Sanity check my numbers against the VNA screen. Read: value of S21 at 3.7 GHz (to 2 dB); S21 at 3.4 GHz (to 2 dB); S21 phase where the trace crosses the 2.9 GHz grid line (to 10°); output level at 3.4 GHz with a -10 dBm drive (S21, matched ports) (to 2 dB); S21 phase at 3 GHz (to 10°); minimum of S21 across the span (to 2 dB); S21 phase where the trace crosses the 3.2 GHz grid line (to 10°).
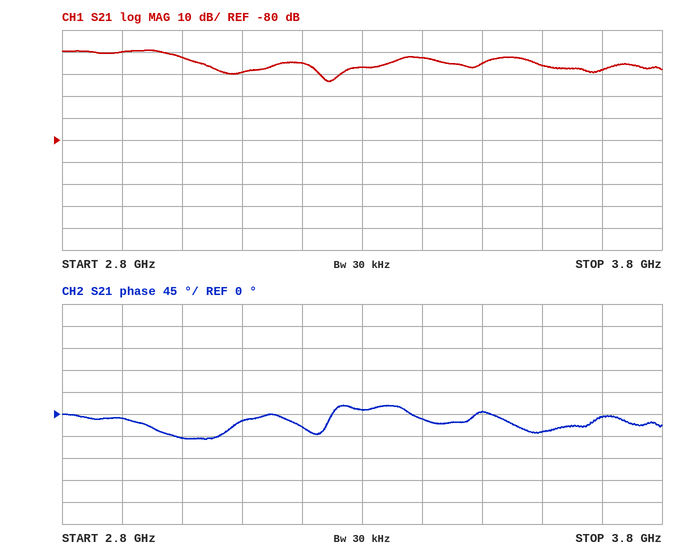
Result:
-48 dB
-42 dB
-10°
-52 dBm
-50°
-54 dB
-30°
